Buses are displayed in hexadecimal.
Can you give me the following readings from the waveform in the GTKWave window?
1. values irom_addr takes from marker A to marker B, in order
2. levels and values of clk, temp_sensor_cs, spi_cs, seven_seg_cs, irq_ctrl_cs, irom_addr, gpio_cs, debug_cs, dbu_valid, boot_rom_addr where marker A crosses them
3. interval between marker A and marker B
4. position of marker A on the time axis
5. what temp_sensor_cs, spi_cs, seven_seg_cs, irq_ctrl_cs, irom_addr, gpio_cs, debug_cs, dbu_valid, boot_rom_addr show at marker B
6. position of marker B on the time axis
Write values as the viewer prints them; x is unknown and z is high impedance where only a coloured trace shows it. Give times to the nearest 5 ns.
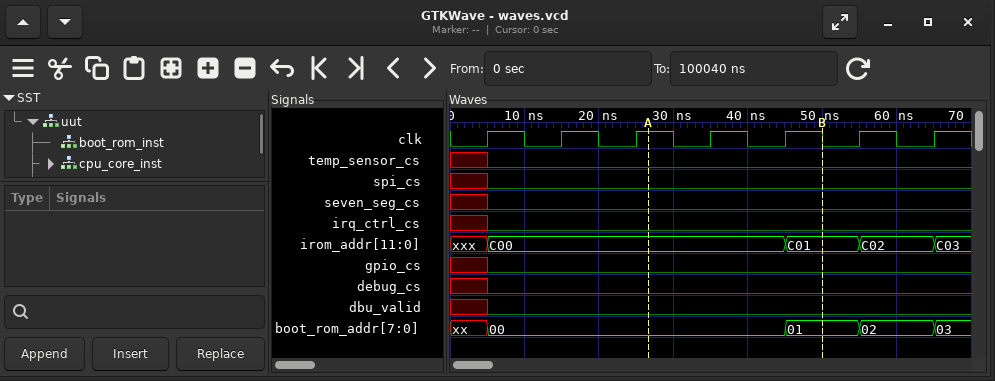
C00, C01
clk=1, temp_sensor_cs=0, spi_cs=0, seven_seg_cs=0, irq_ctrl_cs=0, irom_addr=C00, gpio_cs=0, debug_cs=0, dbu_valid=0, boot_rom_addr=00
25 ns
25 ns
temp_sensor_cs=0, spi_cs=0, seven_seg_cs=0, irq_ctrl_cs=0, irom_addr=C01, gpio_cs=0, debug_cs=0, dbu_valid=0, boot_rom_addr=01
50 ns
